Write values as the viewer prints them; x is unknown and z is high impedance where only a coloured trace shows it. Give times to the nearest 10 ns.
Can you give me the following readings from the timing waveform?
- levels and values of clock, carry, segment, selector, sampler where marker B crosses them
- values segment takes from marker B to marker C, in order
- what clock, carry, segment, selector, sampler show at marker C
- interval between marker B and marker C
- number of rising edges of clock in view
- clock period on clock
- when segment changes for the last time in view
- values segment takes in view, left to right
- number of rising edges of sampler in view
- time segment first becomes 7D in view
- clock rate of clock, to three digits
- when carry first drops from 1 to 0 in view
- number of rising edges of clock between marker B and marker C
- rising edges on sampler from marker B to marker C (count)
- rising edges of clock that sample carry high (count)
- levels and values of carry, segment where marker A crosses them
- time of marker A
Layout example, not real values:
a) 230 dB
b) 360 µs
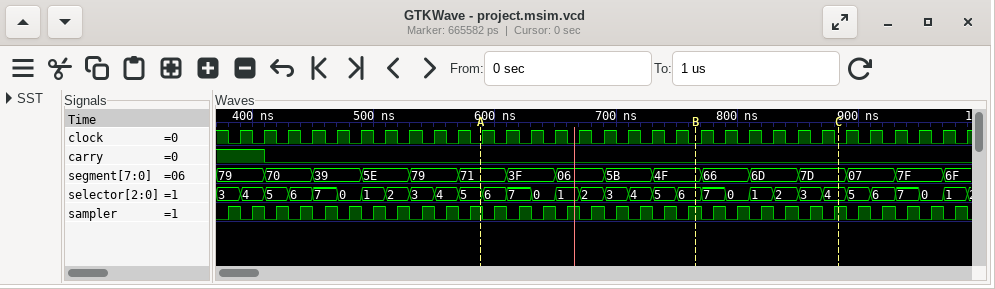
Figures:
a) clock=0, carry=0, segment=4F, selector=6, sampler=1
b) 4F, 66, 6D, 7D
c) clock=0, carry=0, segment=7D, selector=4, sampler=1
d) 120 ns
e) 31
f) 20 ns
g) 970 ns
h) 79, 70, 39, 5E, 79, 71, 3F, 06, 5B, 4F, 66, 6D, 7D, 07, 7F, 6F
i) 31
j) 850 ns
k) 50.0 MHz
l) 410 ns
m) 6
n) 6
o) 2
p) carry=0, segment=71
q) 590 ns
